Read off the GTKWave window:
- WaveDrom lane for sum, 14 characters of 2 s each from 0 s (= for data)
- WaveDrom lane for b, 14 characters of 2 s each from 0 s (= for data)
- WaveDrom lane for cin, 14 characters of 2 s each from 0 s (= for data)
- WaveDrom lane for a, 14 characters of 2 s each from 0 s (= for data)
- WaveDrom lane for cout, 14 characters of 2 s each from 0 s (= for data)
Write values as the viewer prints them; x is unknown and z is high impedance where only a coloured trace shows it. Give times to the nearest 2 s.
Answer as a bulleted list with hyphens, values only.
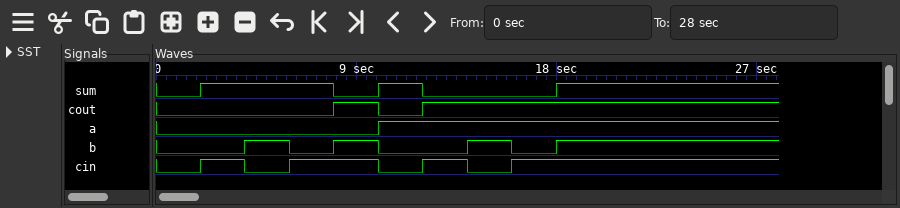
- {name: 'sum', wave: '01..010..1....'}
- {name: 'b', wave: '0.1010.101....'}
- {name: 'cin', wave: '0101.0101.....'}
- {name: 'a', wave: '0....1........'}
- {name: 'cout', wave: '0...101.......'}
